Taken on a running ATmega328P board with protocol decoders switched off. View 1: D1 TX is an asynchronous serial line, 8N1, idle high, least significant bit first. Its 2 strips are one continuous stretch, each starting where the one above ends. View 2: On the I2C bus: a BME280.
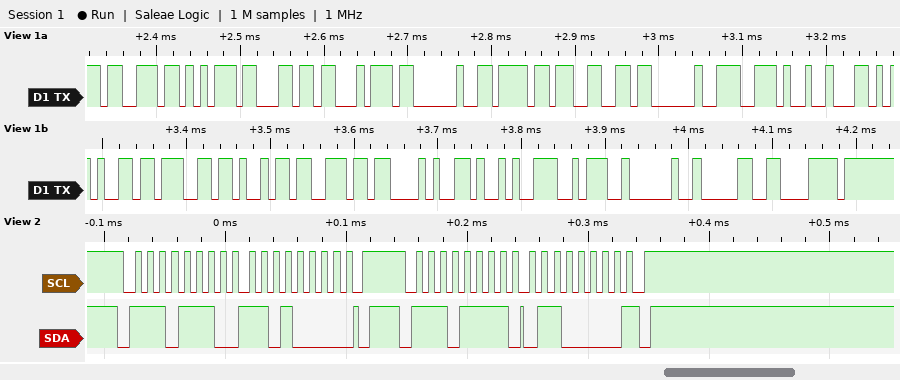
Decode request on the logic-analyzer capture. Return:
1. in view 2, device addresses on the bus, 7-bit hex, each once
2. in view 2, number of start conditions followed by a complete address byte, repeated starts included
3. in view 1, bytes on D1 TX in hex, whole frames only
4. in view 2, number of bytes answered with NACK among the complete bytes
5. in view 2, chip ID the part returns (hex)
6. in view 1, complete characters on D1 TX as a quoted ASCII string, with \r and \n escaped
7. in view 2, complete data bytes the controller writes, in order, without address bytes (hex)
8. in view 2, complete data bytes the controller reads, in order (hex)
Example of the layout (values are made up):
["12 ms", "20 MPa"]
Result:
["0x77", "2", "73 75 6C 74 20 6F 66 20 2E 62 65 67 69 6E 28 29 3A 20 30 78", "1", "0x60", "\"sult of .begin(): 0x\"", "D0", "60"]
